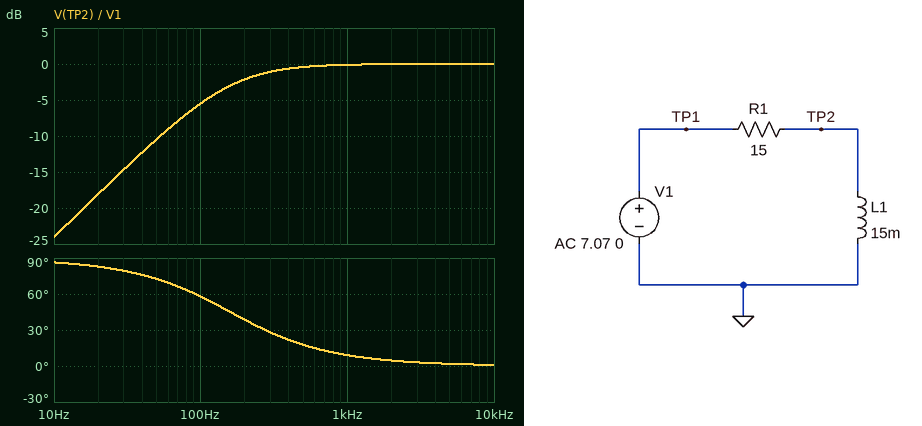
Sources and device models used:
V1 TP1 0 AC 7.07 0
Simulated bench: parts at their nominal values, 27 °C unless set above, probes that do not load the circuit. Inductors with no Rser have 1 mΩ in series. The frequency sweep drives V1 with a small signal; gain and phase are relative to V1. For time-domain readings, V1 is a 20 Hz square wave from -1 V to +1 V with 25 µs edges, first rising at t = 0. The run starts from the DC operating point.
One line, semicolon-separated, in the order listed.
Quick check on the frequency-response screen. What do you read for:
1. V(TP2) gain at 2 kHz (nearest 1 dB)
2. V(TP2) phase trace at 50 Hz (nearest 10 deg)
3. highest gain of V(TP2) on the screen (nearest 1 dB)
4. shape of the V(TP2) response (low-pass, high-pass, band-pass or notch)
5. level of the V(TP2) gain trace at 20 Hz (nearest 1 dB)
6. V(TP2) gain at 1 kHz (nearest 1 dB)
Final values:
0 dB; 70 deg; 0 dB; high-pass; -18 dB; 0 dB
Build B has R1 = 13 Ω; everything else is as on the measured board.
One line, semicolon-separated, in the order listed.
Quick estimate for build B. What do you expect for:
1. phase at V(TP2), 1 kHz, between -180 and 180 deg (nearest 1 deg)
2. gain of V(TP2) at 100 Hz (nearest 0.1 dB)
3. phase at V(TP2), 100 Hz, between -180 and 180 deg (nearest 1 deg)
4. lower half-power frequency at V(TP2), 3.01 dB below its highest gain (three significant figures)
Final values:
8 deg; -4.6 dB; 54 deg; 138 Hz
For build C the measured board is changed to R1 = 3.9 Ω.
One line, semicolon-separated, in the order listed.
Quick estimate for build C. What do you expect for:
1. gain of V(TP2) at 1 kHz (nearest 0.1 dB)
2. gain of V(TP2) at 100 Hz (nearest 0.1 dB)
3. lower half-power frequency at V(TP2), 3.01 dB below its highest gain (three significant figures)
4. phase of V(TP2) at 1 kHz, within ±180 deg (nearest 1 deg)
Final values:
0 dB; -0.7 dB; 41.4 Hz; 2 deg
